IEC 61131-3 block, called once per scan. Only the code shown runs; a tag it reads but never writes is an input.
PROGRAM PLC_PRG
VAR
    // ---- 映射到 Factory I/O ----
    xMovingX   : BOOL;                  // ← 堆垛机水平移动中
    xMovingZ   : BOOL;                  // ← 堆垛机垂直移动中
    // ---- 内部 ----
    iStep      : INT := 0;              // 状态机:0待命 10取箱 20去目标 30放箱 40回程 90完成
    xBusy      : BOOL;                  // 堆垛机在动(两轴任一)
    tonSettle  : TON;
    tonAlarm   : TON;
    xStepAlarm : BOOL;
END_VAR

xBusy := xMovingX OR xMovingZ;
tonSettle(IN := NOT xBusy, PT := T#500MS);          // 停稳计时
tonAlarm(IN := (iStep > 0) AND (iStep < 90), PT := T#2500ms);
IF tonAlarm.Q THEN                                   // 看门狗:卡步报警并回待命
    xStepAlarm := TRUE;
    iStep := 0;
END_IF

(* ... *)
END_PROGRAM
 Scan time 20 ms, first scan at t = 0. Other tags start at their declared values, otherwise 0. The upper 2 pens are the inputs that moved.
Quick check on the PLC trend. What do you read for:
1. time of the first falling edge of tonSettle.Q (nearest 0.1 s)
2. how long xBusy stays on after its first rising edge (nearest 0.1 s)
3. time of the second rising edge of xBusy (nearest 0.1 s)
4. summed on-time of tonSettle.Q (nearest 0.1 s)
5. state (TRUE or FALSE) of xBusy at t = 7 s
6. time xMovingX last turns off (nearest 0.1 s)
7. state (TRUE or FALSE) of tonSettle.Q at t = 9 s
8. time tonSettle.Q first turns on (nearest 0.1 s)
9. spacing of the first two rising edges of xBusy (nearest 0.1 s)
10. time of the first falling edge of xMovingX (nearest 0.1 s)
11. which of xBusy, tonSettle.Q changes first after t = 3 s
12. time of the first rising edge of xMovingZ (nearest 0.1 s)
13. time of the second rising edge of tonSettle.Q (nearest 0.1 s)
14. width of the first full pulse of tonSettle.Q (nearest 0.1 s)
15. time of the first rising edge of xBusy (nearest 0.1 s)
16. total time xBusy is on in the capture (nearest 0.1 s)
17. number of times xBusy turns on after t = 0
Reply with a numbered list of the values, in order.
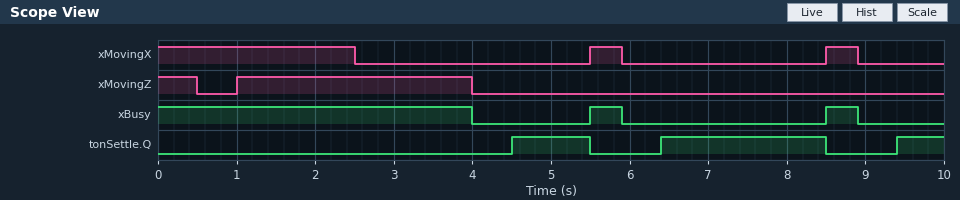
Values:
1. 5.5 s
2. 0.4 s
3. 8.5 s
4. 3.7 s
5. FALSE
6. 8.9 s
7. FALSE
8. 4.5 s
9. 3.0 s
10. 2.5 s
11. xBusy
12. 1.0 s
13. 6.4 s
14. 1.0 s
15. 5.5 s
16. 4.8 s
17. 2
